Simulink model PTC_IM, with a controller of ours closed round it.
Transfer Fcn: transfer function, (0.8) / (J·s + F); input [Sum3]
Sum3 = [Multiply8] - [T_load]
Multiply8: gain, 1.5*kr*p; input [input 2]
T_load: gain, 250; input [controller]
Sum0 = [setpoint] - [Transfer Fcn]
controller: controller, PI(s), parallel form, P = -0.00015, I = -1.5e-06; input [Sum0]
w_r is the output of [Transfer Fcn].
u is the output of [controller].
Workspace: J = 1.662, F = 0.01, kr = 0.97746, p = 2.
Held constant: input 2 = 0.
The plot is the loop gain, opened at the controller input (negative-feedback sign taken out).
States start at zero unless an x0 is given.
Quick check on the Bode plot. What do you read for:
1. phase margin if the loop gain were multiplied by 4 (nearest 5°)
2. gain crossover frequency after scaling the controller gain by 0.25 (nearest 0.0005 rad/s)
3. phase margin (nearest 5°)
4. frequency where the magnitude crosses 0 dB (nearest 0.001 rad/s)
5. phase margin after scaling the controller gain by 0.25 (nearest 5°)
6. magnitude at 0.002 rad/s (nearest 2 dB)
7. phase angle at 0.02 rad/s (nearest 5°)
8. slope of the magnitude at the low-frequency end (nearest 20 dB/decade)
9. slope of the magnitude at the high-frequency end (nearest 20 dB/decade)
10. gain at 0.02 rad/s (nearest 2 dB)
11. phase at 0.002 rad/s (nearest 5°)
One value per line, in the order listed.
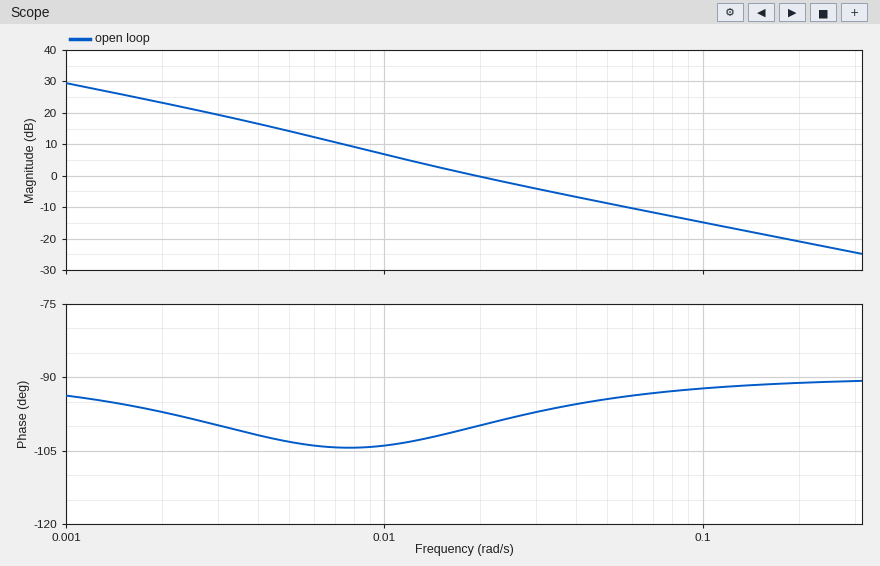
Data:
85°
0.0060 rad/s
80°
0.019 rad/s
75°
24 dB
-100°
-20 dB/decade
-20 dB/decade
0 dB
-95°
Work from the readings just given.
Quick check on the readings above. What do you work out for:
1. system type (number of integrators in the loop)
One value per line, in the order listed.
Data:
1
